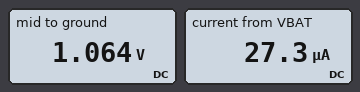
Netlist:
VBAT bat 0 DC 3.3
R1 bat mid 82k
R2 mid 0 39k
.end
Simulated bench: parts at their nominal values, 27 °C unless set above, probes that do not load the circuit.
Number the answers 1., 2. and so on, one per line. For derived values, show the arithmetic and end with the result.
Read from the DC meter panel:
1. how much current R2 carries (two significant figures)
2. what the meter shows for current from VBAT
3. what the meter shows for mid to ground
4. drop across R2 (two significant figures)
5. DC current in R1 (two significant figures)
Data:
1. (1.064 V) / 39 kΩ = 27 µA
2. 27.3 µA
3. 1.064 V
4. 1.064 V = 1.1 V
5. (3.3 V - 1.064 V) / 82 kΩ = 27 µA
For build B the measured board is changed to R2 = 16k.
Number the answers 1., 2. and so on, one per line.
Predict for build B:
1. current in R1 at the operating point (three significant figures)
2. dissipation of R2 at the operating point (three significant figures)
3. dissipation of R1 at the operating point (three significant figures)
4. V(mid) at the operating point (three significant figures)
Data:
1. 33.7 µA
2. 18.1 µW
3. 93.0 µW
4. 539 mV
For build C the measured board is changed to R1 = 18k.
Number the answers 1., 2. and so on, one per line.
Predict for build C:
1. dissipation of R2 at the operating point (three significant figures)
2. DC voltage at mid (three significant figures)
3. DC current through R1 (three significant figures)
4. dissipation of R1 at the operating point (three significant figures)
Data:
1. 131 µW
2. 2.26 V
3. 57.9 µA
4. 60.3 µW
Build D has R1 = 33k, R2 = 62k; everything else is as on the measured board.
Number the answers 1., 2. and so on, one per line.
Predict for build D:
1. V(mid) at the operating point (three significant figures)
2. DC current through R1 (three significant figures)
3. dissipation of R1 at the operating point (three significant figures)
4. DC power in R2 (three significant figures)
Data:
1. 2.15 V
2. 34.7 µA
3. 39.8 µW
4. 74.8 µW
